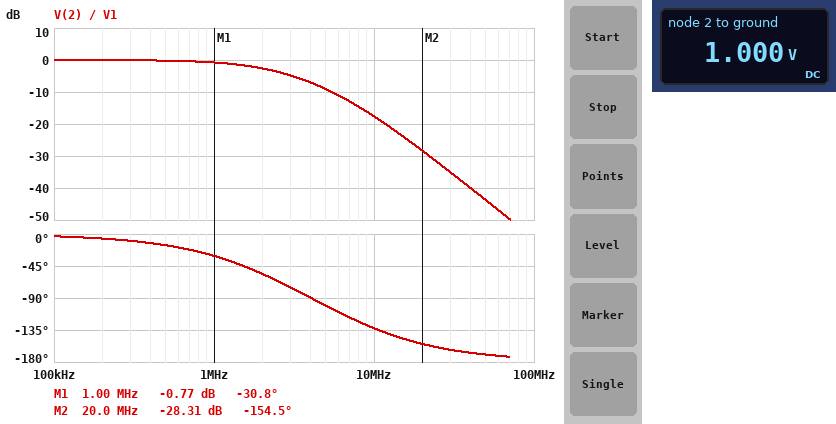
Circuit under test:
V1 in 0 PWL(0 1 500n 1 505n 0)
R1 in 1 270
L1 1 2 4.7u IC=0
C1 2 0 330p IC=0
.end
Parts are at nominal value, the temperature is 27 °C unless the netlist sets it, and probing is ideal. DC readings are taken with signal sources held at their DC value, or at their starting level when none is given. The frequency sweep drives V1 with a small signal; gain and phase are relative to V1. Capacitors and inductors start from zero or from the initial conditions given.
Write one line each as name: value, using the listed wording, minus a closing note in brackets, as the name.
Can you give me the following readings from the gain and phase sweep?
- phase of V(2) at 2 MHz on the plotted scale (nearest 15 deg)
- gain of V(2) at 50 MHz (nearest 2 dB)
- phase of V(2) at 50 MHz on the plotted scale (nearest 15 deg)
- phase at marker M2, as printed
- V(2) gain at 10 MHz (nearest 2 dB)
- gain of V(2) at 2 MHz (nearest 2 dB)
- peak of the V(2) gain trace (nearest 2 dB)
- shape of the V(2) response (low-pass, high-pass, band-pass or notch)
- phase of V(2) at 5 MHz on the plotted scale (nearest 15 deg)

phase of V(2) at 2 MHz on the plotted scale: -60 deg
gain of V(2) at 50 MHz: -44 dB
phase of V(2) at 50 MHz on the plotted scale: -165 deg
phase at marker M2, as printed: -154.5 deg
V(2) gain at 10 MHz: -18 dB
gain of V(2) at 2 MHz: -2 dB
peak of the V(2) gain trace: 0 dB
shape of the V(2) response: low-pass
phase of V(2) at 5 MHz on the plotted scale: -105 deg
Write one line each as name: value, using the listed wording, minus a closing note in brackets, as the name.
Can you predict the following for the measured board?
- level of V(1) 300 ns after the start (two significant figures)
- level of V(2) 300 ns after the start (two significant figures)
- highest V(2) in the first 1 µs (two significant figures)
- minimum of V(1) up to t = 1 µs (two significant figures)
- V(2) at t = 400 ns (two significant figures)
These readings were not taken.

level of V(1) 300 ns after the start: 980 mV
level of V(2) 300 ns after the start: 980 mV
highest V(2) in the first 1 µs: 1.0 V
minimum of V(1) up to t = 1 µs: 1.1 mV
V(2) at t = 400 ns: 1.0 V
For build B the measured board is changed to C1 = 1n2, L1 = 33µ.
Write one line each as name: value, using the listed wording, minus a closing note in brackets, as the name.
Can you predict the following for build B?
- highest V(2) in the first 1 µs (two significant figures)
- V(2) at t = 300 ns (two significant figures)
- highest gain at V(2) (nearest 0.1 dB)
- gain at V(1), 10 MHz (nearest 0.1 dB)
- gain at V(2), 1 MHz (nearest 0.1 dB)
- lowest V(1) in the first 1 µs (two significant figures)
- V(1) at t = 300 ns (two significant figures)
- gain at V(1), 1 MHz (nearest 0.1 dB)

highest V(2) in the first 1 µs: 830 mV
V(2) at t = 300 ns: 500 mV
highest gain at V(2): 0 dB
gain at V(1), 10 MHz: -0.1 dB
gain at V(2), 1 MHz: -6.5 dB
lowest V(1) in the first 1 µs: -330 mV
V(1) at t = 300 ns: 370 mV
gain at V(1), 1 MHz: -11.5 dB
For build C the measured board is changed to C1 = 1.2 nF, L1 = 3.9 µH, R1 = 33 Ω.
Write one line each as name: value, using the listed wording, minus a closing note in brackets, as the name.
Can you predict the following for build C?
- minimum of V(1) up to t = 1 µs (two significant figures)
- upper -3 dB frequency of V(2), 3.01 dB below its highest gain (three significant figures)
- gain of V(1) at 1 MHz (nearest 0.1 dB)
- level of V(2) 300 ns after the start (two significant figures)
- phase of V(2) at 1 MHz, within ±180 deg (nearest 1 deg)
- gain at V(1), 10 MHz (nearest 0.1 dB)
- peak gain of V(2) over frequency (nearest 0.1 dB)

minimum of V(1) up to t = 1 µs: -140 mV
upper -3 dB frequency of V(2), 3.01 dB below its highest gain: 2.74 MHz
gain of V(1) at 1 MHz: -0.4 dB
level of V(2) 300 ns after the start: 1.2 V
phase of V(2) at 1 MHz, within ±180 deg: -17 deg
gain at V(1), 10 MHz: -0.1 dB
peak gain of V(2) over frequency: 5.1 dB
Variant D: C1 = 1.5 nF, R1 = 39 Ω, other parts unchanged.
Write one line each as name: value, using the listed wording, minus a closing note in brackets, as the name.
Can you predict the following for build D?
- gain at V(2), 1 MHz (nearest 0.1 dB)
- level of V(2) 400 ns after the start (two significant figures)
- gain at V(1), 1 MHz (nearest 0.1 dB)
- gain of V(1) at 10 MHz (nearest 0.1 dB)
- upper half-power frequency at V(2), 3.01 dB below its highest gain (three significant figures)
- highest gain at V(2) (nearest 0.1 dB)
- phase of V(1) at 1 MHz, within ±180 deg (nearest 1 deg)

gain at V(2), 1 MHz: 1.8 dB
level of V(2) 400 ns after the start: 1.1 V
gain at V(1), 1 MHz: -1.0 dB
gain of V(1) at 10 MHz: -0.1 dB
upper half-power frequency at V(2), 3.01 dB below its highest gain: 2.25 MHz
highest gain at V(2): 3.7 dB
phase of V(1) at 1 MHz, within ±180 deg: -27 deg
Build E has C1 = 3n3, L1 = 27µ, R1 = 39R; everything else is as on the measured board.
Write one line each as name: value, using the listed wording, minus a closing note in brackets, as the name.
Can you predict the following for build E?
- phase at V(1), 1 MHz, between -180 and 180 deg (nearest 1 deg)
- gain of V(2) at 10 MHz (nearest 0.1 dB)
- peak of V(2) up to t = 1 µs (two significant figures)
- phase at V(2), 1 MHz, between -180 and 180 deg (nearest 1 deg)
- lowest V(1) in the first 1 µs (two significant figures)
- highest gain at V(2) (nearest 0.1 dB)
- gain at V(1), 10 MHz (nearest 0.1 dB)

phase at V(1), 1 MHz, between -180 and 180 deg: 18 deg
gain of V(2) at 10 MHz: -50.9 dB
peak of V(2) up to t = 1 µs: 1.1 V
phase at V(2), 1 MHz, between -180 and 180 deg: -162 deg
lowest V(1) in the first 1 µs: -300 mV
highest gain at V(2): 7.5 dB
gain at V(1), 10 MHz: 0 dB
